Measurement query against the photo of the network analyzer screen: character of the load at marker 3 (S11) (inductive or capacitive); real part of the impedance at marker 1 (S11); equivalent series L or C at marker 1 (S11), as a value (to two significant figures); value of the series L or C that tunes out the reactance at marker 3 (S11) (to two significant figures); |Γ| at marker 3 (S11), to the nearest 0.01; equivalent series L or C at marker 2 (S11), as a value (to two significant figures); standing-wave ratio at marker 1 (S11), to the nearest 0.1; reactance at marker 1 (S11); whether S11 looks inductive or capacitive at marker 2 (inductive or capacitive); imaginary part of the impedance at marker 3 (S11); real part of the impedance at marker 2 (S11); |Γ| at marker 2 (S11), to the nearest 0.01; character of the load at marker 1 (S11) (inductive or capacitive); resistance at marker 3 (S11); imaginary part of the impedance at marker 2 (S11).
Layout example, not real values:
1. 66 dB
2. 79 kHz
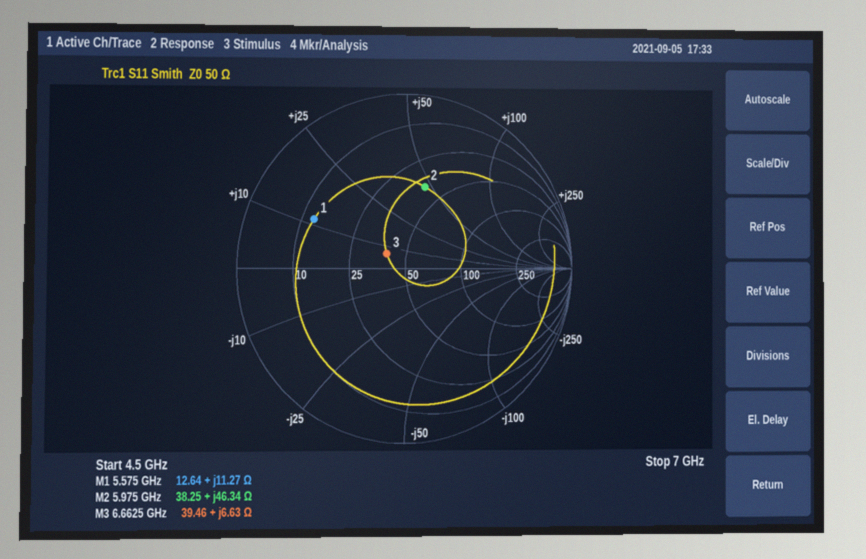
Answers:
1. inductive
2. 12.64 Ω
3. 320 pH
4. 3.6 pF
5. 0.14
6. 1.2 nH
7. 4.2
8. +11.27 Ω
9. inductive
10. +6.63 Ω
11. 38.25 Ω
12. 0.48
13. inductive
14. 39.46 Ω
15. +46.34 Ω
